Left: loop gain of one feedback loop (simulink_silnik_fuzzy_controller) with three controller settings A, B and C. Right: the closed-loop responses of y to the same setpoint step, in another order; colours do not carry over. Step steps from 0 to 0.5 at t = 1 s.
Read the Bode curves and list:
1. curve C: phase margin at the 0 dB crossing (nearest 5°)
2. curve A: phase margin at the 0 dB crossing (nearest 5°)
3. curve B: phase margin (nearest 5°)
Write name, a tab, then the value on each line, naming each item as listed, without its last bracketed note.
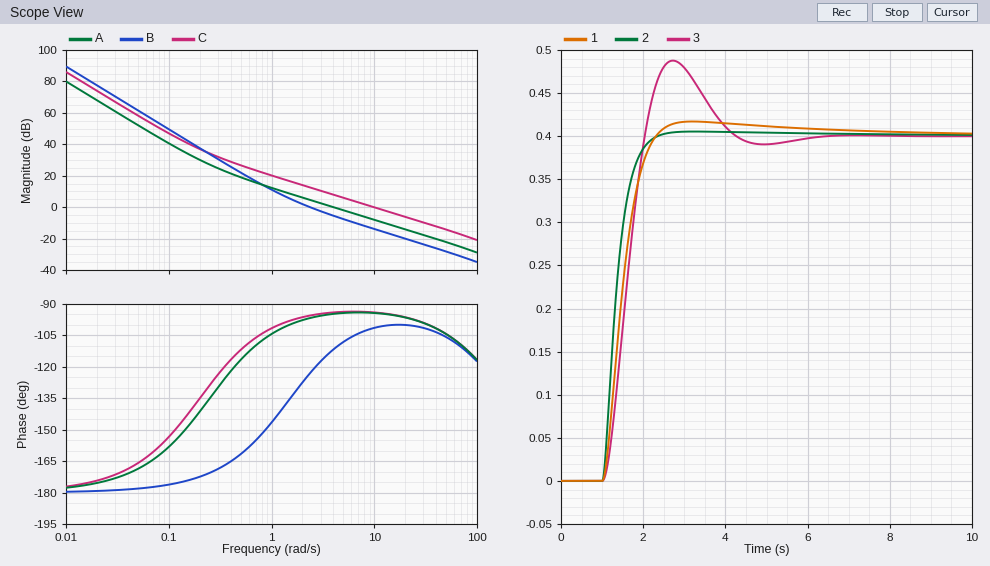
curve C: phase margin at the 0 dB crossing	85°
curve A: phase margin at the 0 dB crossing	85°
curve B: phase margin	55°
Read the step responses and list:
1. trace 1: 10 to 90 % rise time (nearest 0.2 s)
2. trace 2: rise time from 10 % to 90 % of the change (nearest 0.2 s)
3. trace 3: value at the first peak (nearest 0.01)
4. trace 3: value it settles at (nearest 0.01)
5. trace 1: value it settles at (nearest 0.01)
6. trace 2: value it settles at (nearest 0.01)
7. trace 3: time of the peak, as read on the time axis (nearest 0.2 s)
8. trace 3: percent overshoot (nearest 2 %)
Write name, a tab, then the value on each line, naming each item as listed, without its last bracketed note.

trace 1: 10 to 90 % rise time	0.8 s
trace 2: rise time from 10 % to 90 % of the change	0.6 s
trace 3: value at the first peak	0.49
trace 3: value it settles at	0.40
trace 1: value it settles at	0.40
trace 2: value it settles at	0.40
trace 3: time of the peak, as read on the time axis	2.8 s
trace 3: percent overshoot	22 %
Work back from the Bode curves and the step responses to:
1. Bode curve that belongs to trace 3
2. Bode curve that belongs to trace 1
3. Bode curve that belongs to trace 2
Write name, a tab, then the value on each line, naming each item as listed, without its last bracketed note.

Bode curve that belongs to trace 3	B
Bode curve that belongs to trace 1	A
Bode curve that belongs to trace 2	C
